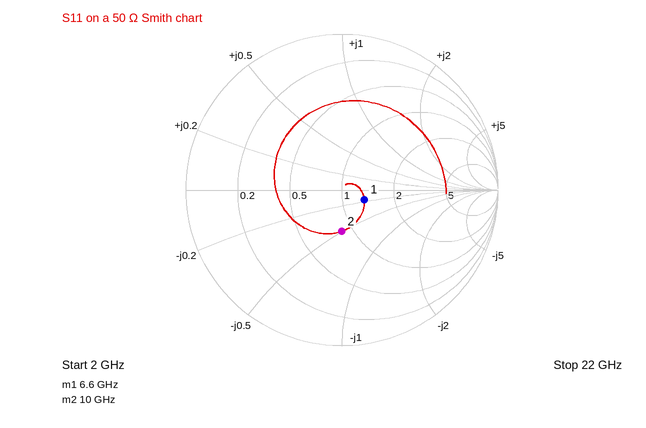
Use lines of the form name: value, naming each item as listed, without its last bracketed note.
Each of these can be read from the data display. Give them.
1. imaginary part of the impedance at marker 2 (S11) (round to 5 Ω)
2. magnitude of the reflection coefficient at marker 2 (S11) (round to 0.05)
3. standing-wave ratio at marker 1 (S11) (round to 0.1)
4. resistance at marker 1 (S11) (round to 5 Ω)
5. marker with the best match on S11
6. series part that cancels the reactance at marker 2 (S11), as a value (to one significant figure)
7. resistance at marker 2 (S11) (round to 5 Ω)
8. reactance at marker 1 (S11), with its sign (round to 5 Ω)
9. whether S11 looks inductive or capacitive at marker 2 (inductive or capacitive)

imaginary part of the impedance at marker 2 (S11): -25 Ω
magnitude of the reflection coefficient at marker 2 (S11): 0.25
standing-wave ratio at marker 1 (S11): 1.4
resistance at marker 1 (S11): 65 Ω
marker with the best match on S11: marker 1
series part that cancels the reactance at marker 2 (S11), as a value: 400 pH
resistance at marker 2 (S11): 45 Ω
reactance at marker 1 (S11), with its sign: -10 Ω
whether S11 looks inductive or capacitive at marker 2: capacitive
